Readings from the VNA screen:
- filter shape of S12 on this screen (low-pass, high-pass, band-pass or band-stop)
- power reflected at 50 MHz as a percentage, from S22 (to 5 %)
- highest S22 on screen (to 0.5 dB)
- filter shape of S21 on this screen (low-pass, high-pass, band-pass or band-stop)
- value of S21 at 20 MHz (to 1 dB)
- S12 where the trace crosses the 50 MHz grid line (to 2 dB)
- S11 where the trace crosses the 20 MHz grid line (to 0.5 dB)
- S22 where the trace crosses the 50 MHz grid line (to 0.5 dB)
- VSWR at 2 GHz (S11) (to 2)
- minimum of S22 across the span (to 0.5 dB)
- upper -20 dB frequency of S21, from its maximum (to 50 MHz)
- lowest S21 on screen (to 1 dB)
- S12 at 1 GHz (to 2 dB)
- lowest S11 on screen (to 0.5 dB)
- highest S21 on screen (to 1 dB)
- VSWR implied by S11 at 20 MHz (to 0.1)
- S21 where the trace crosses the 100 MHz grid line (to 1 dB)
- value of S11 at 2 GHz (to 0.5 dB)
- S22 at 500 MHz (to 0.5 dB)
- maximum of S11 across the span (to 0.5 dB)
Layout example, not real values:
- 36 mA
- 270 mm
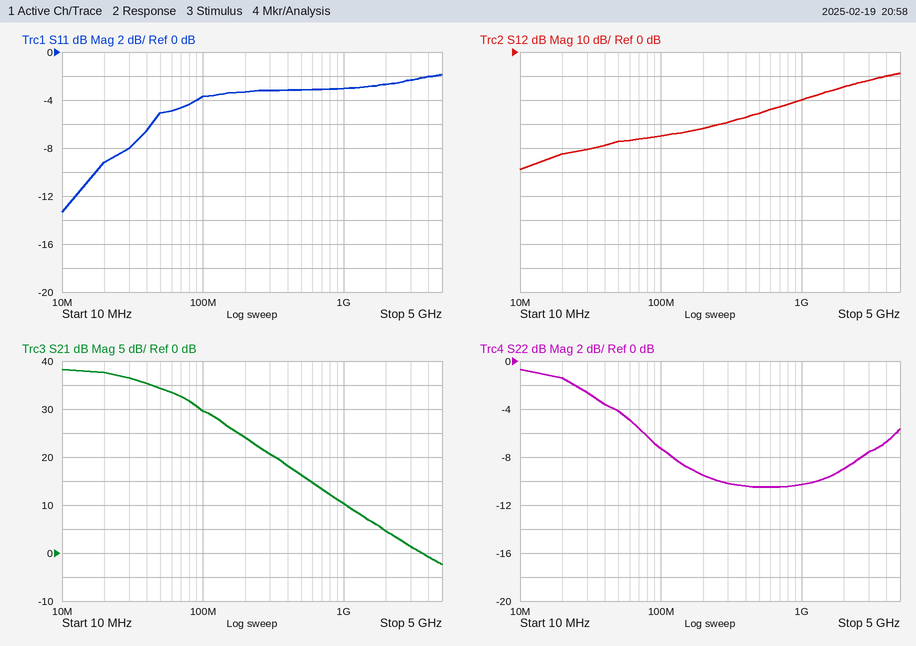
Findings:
- high-pass
- 40 %
- -0.5 dB
- low-pass
- 38 dB
- -38 dB
- -9.0 dB
- -4.0 dB
- 6
- -10.5 dB
- 400 MHz
- -2 dB
- -20 dB
- -13.5 dB
- 38 dB
- 2.1
- 30 dB
- -2.5 dB
- -10.5 dB
- -2.0 dB
